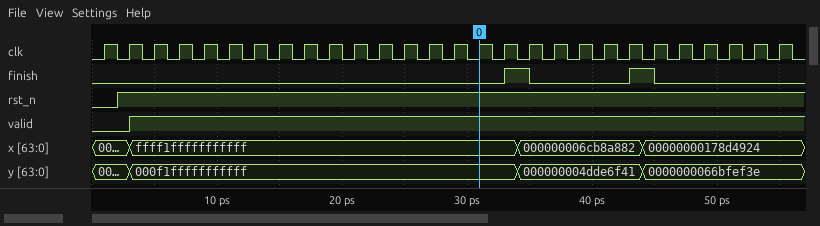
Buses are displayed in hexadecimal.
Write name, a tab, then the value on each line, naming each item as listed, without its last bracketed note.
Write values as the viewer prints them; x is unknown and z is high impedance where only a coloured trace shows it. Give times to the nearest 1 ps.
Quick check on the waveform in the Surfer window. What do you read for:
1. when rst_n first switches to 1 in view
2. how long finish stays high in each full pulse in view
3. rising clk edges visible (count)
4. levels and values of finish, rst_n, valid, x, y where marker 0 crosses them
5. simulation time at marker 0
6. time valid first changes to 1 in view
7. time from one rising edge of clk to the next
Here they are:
when rst_n first switches to 1 in view	2 ps
how long finish stays high in each full pulse in view	2 ps, 2 ps
rising clk edges visible	28
levels and values of finish, rst_n, valid, x, y where marker 0 crosses them	finish=0, rst_n=1, valid=1, x=ffff1fffffffffff, y=000f1fffffffffff
simulation time at marker 0	31 ps
time valid first changes to 1 in view	3 ps
time from one rising edge of clk to the next	2 ps
